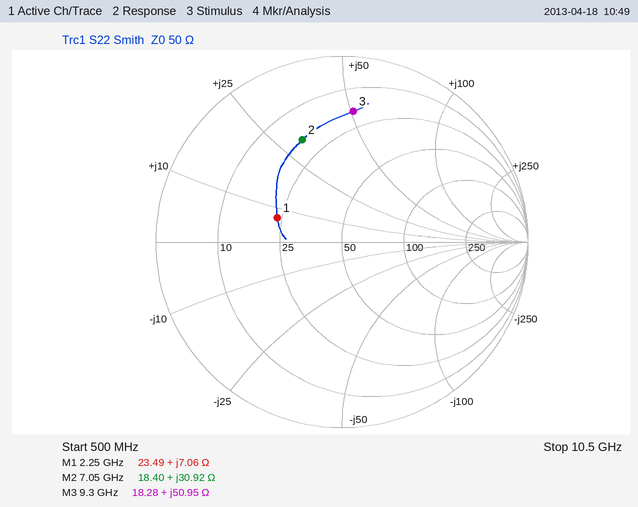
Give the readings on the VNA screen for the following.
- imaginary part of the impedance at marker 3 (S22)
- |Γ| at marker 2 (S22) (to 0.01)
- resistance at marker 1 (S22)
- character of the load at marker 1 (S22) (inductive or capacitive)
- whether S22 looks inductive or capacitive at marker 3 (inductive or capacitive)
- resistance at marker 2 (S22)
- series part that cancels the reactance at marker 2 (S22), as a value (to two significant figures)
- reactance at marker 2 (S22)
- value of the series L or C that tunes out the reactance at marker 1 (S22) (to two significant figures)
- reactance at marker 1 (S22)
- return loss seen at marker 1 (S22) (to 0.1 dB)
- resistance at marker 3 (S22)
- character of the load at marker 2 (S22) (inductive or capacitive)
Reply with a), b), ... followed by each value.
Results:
a) +50.95 Ω
b) 0.59
c) 23.49 Ω
d) inductive
e) inductive
f) 18.40 Ω
g) 730 fF
h) +30.92 Ω
i) 10 pF
j) +7.06 Ω
k) 8.6 dB
l) 18.28 Ω
m) inductive
